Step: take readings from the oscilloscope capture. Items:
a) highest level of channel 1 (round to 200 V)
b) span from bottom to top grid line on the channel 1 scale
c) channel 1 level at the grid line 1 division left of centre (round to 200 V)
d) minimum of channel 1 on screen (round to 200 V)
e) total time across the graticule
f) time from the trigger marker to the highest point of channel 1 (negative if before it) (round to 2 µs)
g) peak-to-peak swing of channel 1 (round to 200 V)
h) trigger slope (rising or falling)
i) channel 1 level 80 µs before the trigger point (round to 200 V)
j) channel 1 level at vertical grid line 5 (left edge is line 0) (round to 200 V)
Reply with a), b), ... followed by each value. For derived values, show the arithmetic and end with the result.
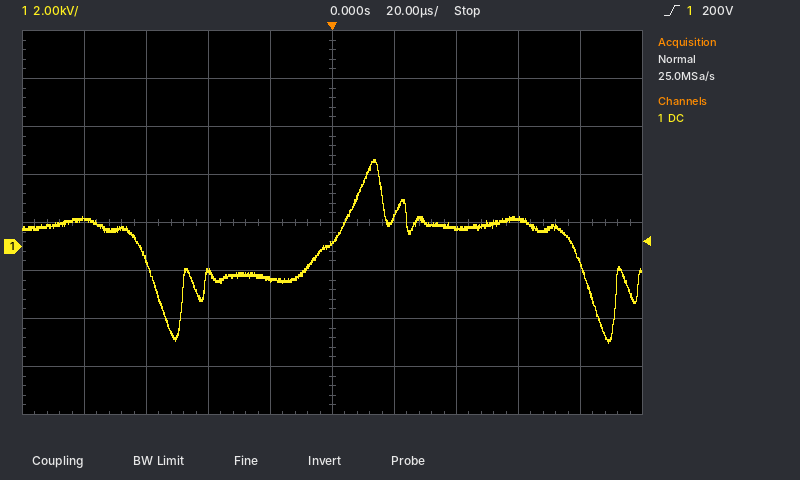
a) 3.6 kV
b) 16 kV
c) -1.4 kV
d) -4.0 kV
e) 200 µs
f) +14 µs
g) 3.6 kV − (-4.0 kV) = 7.6 kV
h) rising
i) 1.2 kV
j) 200 V
